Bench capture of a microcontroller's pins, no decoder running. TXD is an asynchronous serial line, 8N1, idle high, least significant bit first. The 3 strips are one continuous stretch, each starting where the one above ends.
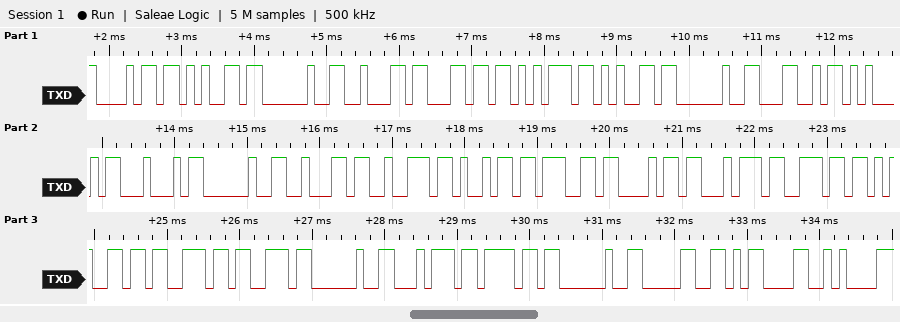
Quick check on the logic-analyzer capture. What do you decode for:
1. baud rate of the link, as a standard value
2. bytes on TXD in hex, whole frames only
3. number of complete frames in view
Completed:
9600 baud
68 65 20 62 6C 75 65 20 4C 45 44 20 62 72 69 67 68 74 6E 65 73 73 20 74 6F 20 30 0D 0A
29
